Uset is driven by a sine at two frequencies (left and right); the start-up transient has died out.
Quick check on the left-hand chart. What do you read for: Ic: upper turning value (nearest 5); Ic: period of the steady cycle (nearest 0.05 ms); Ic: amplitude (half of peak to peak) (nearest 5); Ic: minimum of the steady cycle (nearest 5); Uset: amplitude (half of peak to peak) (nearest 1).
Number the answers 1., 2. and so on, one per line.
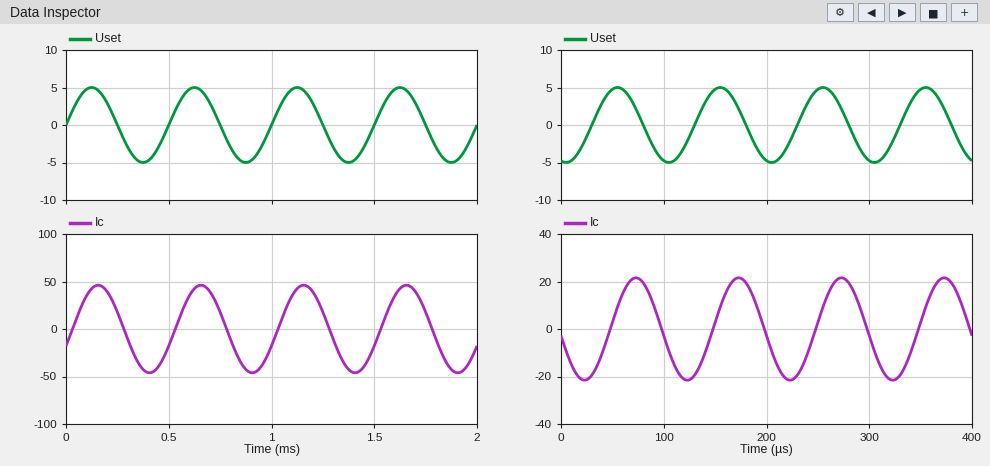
1. 45
2. 0.50 ms
3. 45
4. -45
5. 5
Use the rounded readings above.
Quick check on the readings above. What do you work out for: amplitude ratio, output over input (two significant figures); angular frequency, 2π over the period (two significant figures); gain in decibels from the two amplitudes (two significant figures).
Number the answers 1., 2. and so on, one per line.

1. 9.0
2. 13 rad/ms
3. 19 dB
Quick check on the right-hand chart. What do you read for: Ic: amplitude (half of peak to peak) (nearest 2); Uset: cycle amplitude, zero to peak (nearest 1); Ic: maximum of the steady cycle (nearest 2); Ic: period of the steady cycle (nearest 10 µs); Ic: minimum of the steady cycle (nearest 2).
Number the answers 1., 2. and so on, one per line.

1. 22
2. 5
3. 22
4. 100 µs
5. -22
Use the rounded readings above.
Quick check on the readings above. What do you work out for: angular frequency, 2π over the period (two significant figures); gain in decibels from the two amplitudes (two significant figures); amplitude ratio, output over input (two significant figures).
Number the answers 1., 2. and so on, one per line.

1. 0.063 rad/µs
2. 13 dB
3. 4.4
